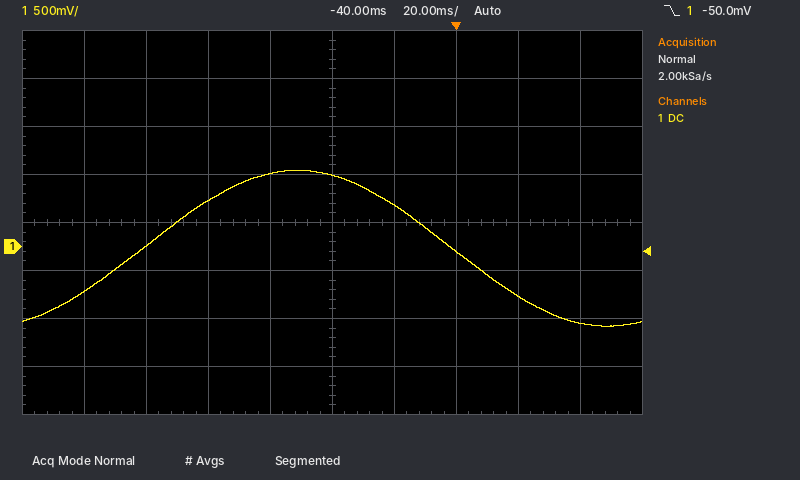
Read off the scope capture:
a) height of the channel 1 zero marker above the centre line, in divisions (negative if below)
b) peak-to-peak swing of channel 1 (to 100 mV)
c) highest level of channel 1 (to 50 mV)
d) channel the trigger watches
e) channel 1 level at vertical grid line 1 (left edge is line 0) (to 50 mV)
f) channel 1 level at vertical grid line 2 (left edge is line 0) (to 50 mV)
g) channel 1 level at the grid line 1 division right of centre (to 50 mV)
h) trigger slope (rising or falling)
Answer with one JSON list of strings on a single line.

["-0.5 div", "1.60 V", "800 mV", "channel 1", "-450 mV", "0 mV", "450 mV", "falling"]
